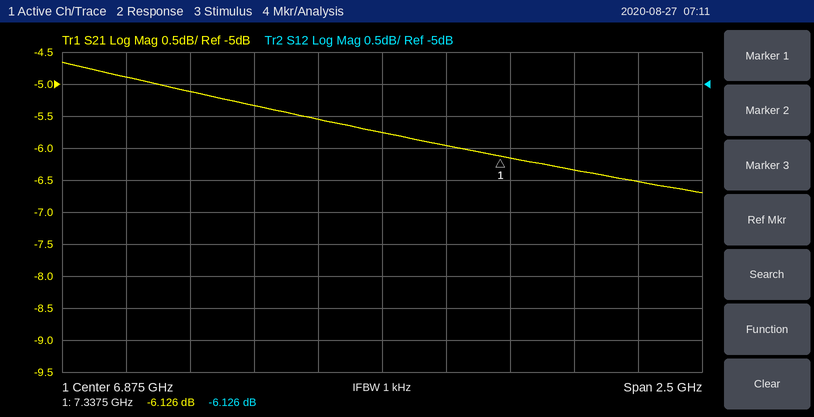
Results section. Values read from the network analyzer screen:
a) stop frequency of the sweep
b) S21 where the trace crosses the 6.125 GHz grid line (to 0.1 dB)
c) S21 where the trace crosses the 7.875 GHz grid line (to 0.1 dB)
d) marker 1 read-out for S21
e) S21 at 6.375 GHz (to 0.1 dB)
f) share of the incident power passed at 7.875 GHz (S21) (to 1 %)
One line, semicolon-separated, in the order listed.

8.125 GHz; -5.1 dB; -6.5 dB; -6.126 dB; -5.3 dB; 22 %
